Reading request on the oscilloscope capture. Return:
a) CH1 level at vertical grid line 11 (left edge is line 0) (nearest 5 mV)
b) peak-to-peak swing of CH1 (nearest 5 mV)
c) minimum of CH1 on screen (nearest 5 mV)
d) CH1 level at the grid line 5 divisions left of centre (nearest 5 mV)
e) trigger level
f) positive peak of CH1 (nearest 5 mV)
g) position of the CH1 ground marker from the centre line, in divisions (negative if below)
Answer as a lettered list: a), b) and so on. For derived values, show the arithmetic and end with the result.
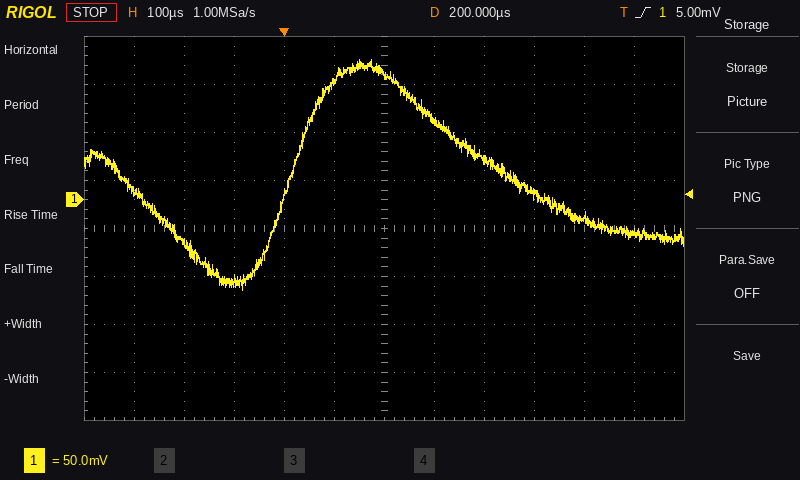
a) -35 mV
b) 145 mV − (-95 mV) = 240 mV
c) -95 mV
d) 10 mV
e) 5.00 mV
f) 145 mV
g) +0.6 div
